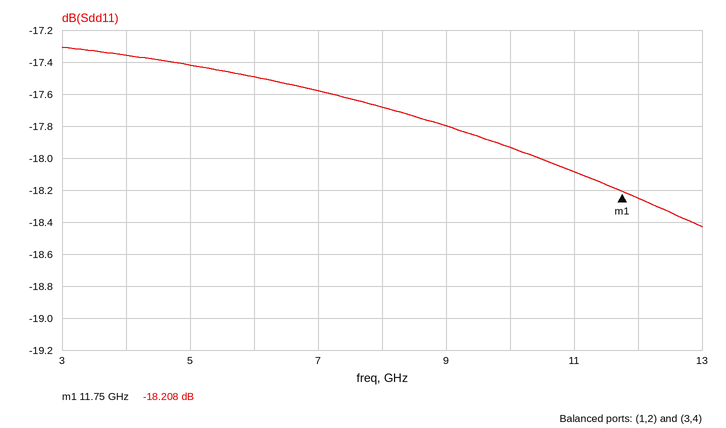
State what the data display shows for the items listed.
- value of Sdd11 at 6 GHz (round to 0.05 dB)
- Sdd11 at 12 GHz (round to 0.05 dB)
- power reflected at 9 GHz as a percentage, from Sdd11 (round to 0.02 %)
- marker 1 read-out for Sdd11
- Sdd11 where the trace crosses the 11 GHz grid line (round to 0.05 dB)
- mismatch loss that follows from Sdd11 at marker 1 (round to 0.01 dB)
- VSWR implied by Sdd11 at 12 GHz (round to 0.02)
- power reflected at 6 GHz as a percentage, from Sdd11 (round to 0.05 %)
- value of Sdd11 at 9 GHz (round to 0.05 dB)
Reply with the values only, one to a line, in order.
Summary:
-17.50 dB
-18.25 dB
1.66 %
-18.208 dB
-18.10 dB
0.07 dB
1.28
1.80 %
-17.80 dB
